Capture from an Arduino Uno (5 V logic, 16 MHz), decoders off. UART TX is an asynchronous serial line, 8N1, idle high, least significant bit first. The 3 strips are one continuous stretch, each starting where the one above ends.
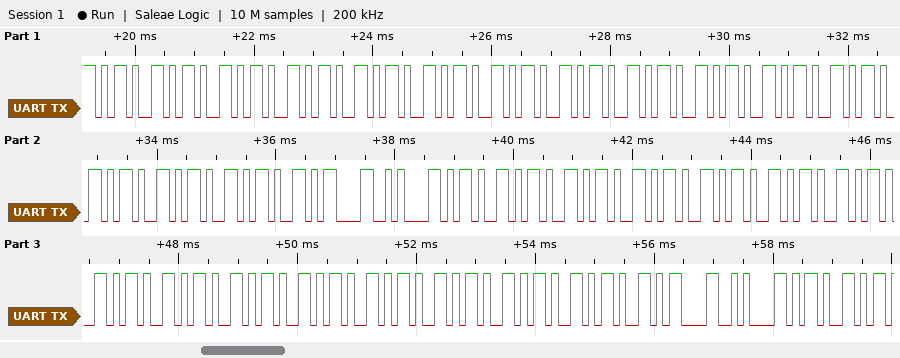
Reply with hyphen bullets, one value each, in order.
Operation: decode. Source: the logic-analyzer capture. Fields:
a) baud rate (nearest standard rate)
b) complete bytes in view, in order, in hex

- 9600 baud
- 2D 2D 2D 2D 2D 2D 2D 2D 2D 2D 2D 2D 2D 2D 2D 0D 0A 2D 2D 2D 2D 2D 2D 2D 2D 2D 2D 2D 2D 2D 2D 2D 0D 0A 2D
